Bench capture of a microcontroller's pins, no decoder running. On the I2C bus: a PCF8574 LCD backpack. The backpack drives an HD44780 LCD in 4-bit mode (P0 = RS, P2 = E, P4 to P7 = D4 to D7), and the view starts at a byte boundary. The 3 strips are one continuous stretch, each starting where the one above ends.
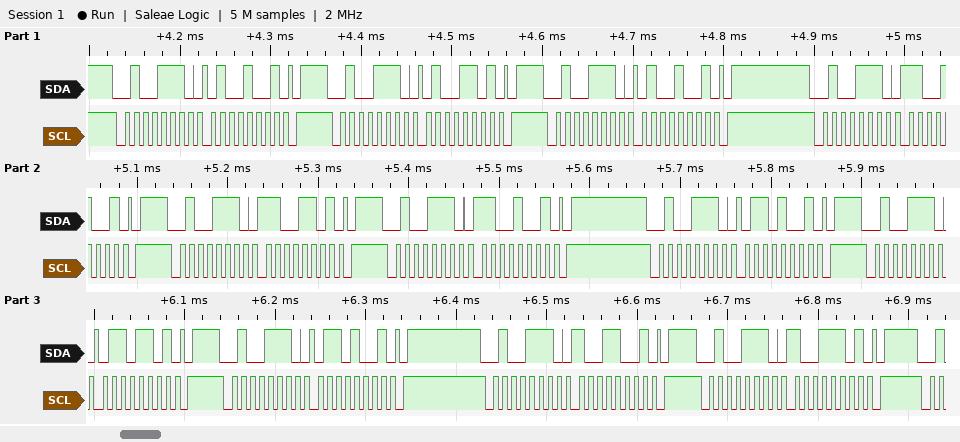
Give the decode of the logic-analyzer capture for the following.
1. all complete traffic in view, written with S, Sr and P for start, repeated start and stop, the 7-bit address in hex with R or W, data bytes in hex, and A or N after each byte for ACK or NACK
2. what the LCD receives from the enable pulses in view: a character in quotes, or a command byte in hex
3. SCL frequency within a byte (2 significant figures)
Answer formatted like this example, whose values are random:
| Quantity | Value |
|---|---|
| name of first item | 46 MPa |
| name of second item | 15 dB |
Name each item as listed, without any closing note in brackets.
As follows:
| Quantity | Value |
|---|---|
| all complete traffic in view, written with S, Sr and P for start, repeated start and stop, the 7-bit address in hex with R or W, data bytes in hex, and A or N after each byte for ACK or NACK | S 27W A 49 A P S 27W A 4D A P S 27W A 49 A P S 27W A C9 A P S 27W A CD A P S 27W A C9 A P S 27W A 69 A P S 27W A 6D A P S 27W A 69 A P S 27W A 99 A P S 27W A 9D A P |
| what the LCD receives from the enable pulses in view: a character in quotes, or a command byte in hex | 'L' |
| SCL frequency within a byte | 100 kHz |
